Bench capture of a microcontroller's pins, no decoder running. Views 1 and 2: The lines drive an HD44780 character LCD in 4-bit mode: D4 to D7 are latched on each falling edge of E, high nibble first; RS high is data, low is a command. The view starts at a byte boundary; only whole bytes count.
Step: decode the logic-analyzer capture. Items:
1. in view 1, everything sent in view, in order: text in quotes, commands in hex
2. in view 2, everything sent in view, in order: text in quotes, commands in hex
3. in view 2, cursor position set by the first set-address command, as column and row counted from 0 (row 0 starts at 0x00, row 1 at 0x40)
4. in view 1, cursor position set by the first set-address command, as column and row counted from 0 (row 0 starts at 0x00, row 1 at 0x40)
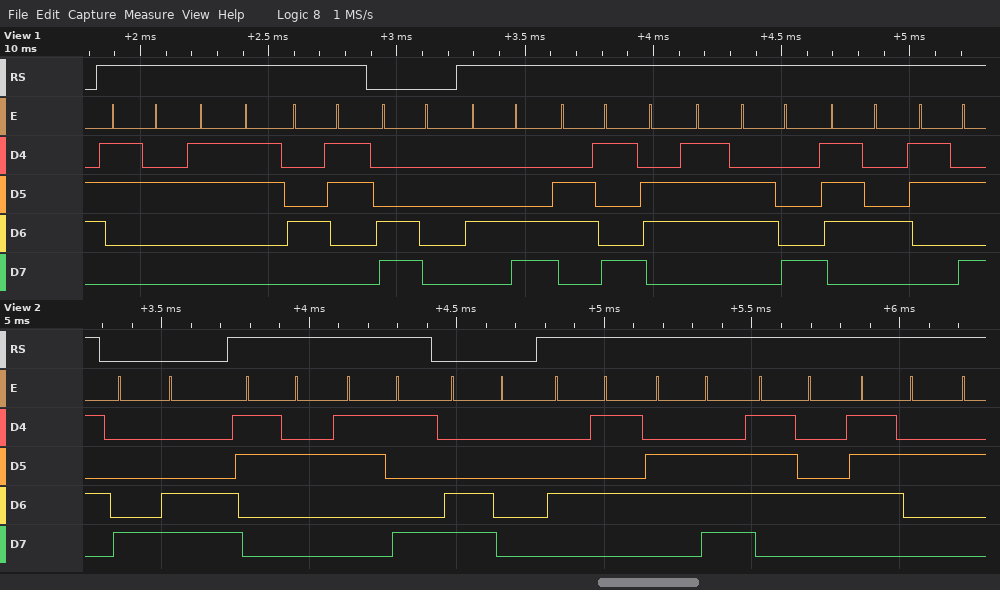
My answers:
"23C" 0xC0 "Light:"
0x8C "29" 0xC0 "Entr"
column 12, row 0
column 0, row 1
